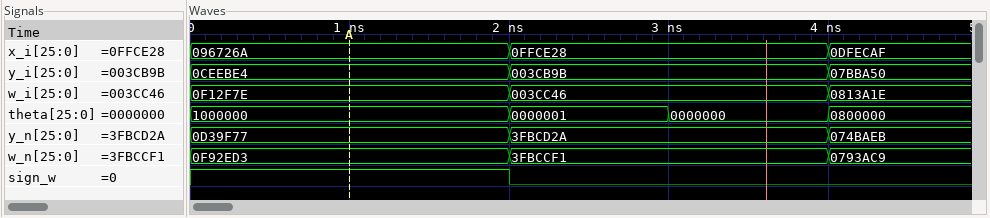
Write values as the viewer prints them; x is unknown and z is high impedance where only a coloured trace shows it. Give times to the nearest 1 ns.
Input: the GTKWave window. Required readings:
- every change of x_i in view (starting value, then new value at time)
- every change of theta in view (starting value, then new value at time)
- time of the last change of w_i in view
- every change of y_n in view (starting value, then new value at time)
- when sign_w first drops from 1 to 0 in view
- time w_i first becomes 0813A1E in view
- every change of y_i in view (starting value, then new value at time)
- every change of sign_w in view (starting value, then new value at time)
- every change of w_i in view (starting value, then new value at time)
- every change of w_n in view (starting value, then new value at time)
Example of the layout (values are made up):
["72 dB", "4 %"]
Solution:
["096726A, 0FFCE28 at 2 ns, 0DFECAF at 4 ns", "1000000, 0000001 at 2 ns, 0000000 at 3 ns, 0800000 at 4 ns", "4 ns", "0D39F77, 3FBCD2A at 2 ns, 074BAEB at 4 ns", "2 ns", "4 ns", "0CEEBE4, 003CB9B at 2 ns, 07BBA50 at 4 ns", "1, 0 at 2 ns", "0F12F7E, 003CC46 at 2 ns, 0813A1E at 4 ns", "0F92ED3, 3FBCCF1 at 2 ns, 0793AC9 at 4 ns"]
